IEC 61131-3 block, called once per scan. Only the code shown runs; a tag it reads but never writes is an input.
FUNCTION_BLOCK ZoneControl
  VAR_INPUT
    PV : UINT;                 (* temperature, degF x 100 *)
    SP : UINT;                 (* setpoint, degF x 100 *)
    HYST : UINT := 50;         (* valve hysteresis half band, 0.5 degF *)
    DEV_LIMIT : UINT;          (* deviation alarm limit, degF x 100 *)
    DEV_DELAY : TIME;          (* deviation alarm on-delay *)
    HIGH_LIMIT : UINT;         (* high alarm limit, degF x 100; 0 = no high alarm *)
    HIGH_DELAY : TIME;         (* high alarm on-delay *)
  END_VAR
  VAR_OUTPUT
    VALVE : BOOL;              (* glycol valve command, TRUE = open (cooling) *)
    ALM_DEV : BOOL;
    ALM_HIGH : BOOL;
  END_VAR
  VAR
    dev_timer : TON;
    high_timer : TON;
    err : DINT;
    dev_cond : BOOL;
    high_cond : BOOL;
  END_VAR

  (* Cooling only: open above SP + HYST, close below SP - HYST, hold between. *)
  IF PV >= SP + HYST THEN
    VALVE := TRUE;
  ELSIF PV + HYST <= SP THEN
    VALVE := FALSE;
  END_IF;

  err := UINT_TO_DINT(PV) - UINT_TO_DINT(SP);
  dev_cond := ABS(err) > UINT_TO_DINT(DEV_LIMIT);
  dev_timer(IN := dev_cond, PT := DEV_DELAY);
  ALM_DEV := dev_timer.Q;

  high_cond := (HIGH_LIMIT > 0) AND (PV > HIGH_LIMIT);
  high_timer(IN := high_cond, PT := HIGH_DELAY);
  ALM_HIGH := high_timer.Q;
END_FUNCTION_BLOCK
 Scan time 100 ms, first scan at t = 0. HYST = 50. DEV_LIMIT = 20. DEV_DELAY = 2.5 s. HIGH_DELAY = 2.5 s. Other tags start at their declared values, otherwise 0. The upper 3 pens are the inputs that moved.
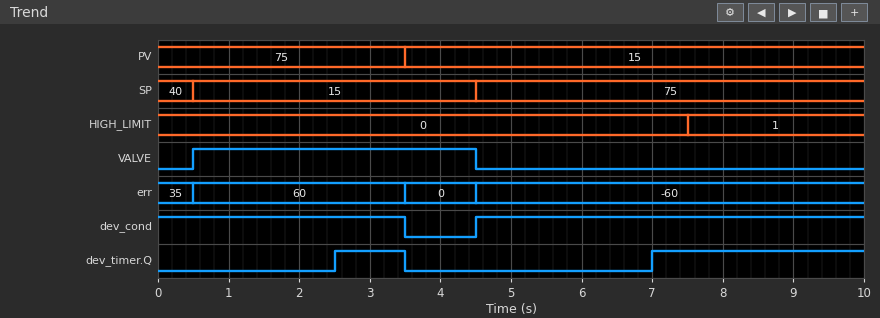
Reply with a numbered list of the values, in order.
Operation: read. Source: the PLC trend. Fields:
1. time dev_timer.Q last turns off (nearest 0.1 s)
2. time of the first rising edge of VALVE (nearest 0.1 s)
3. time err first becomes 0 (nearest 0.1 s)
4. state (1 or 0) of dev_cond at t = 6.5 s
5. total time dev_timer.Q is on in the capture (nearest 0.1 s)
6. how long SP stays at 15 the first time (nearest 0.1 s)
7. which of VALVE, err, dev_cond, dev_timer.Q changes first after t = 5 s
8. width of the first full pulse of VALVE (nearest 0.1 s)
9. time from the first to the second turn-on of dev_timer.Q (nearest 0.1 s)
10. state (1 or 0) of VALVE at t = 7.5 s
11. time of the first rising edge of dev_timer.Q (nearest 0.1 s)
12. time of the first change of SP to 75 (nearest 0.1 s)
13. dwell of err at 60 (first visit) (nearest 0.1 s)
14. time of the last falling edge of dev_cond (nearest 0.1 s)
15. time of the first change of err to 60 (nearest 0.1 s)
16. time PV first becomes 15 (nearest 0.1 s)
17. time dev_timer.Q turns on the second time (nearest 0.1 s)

1. 3.5 s
2. 0.5 s
3. 3.5 s
4. 1
5. 4.0 s
6. 4.0 s
7. dev_timer.Q
8. 4.0 s
9. 4.5 s
10. 0
11. 2.5 s
12. 4.5 s
13. 3.0 s
14. 3.5 s
15. 0.5 s
16. 3.5 s
17. 7.0 s
